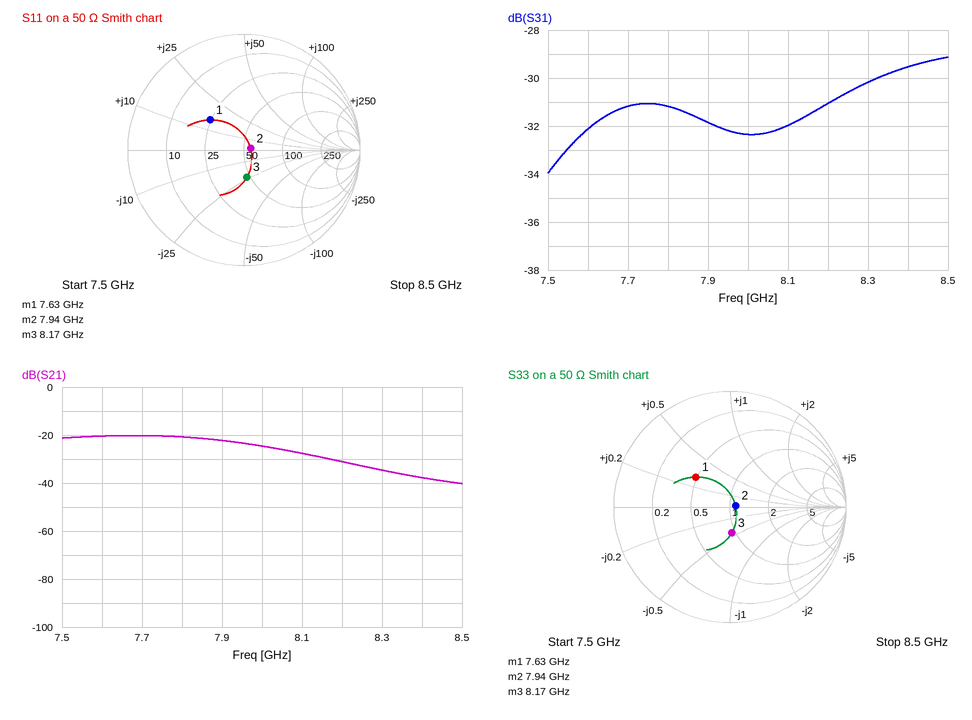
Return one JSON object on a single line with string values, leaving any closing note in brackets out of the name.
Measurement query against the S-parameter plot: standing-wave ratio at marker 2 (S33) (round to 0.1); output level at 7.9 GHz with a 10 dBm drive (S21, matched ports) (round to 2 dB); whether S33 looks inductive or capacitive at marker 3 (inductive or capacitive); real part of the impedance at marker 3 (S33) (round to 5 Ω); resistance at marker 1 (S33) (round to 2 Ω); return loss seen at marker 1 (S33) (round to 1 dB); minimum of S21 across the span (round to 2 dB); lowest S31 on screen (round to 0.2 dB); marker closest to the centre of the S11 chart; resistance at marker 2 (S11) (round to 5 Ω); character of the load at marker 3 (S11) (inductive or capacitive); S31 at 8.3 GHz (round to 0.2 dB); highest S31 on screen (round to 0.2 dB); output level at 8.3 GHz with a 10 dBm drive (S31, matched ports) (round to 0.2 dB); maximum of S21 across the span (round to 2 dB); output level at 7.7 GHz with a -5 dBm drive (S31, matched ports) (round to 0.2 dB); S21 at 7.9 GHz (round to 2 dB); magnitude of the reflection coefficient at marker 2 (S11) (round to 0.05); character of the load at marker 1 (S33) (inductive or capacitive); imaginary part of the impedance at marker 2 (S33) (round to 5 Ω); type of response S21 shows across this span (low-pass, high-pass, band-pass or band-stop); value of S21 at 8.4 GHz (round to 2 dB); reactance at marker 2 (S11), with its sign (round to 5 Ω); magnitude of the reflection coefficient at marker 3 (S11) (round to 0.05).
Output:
{"standing-wave ratio at marker 2 (S33)": "1.1", "output level at 7.9 GHz with a 10 dBm drive (S21, matched ports)": "-12 dBm", "whether S33 looks inductive or capacitive at marker 3": "capacitive", "real part of the impedance at marker 3 (S33)": "45 Ω", "resistance at marker 1 (S33)": "24 Ω", "return loss seen at marker 1 (S33)": "8 dB", "minimum of S21 across the span": "-40 dB", "lowest S31 on screen": "-34.0 dB", "marker closest to the centre of the S11 chart": "marker 2", "resistance at marker 2 (S11)": "55 Ω", "character of the load at marker 3 (S11)": "capacitive", "S31 at 8.3 GHz": "-30.2 dB", "highest S31 on screen": "-29.2 dB", "output level at 8.3 GHz with a 10 dBm drive (S31, matched ports)": "-20.2 dBm", "maximum of S21 across the span": "-20 dB", "output level at 7.7 GHz with a -5 dBm drive (S31, matched ports)": "-36.2 dBm", "S21 at 7.9 GHz": "-22 dB", "magnitude of the reflection coefficient at marker 2 (S11)": "0.05", "character of the load at marker 1 (S33)": "inductive", "imaginary part of the impedance at marker 2 (S33)": "0 Ω", "type of response S21 shows across this span": "low-pass", "value of S21 at 8.4 GHz": "-38 dB", "reactance at marker 2 (S11), with its sign": "0 Ω", "magnitude of the reflection coefficient at marker 3 (S11)": "0.25"}
